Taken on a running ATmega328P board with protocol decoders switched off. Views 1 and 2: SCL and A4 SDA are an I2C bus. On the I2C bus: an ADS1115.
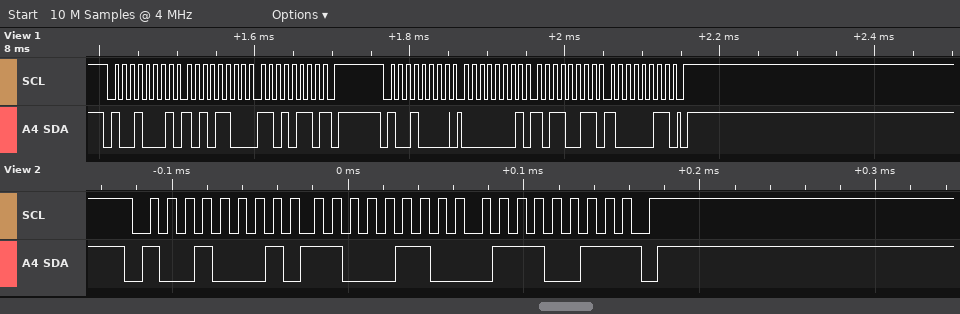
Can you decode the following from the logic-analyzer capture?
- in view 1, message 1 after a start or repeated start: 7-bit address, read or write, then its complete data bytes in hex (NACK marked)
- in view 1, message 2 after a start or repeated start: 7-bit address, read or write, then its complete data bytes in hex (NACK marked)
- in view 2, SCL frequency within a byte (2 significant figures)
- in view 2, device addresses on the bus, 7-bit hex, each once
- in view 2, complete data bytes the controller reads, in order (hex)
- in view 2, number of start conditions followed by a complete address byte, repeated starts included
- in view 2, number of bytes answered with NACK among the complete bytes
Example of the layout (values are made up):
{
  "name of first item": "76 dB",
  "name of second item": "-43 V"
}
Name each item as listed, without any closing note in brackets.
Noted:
{
  "in view 1, message 1 after a start or repeated start: 7-bit address, read or write, then its complete data bytes in hex": "0x48 read: AC D6 NACK",
  "in view 1, message 2 after a start or repeated start: 7-bit address, read or write, then its complete data bytes in hex": "0x48 write: 01 B3 83",
  "in view 2, SCL frequency within a byte": "100 kHz",
  "in view 2, device addresses on the bus, 7-bit hex, each once": "0x48",
  "in view 2, complete data bytes the controller reads, in order": "C6 73",
  "in view 2, number of start conditions followed by a complete address byte, repeated starts included": "1",
  "in view 2, number of bytes answered with NACK among the complete bytes": "1"
}
